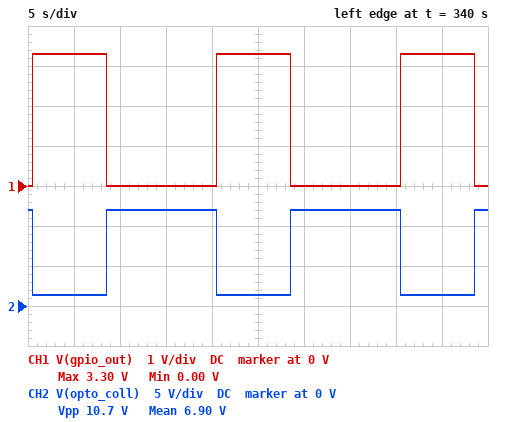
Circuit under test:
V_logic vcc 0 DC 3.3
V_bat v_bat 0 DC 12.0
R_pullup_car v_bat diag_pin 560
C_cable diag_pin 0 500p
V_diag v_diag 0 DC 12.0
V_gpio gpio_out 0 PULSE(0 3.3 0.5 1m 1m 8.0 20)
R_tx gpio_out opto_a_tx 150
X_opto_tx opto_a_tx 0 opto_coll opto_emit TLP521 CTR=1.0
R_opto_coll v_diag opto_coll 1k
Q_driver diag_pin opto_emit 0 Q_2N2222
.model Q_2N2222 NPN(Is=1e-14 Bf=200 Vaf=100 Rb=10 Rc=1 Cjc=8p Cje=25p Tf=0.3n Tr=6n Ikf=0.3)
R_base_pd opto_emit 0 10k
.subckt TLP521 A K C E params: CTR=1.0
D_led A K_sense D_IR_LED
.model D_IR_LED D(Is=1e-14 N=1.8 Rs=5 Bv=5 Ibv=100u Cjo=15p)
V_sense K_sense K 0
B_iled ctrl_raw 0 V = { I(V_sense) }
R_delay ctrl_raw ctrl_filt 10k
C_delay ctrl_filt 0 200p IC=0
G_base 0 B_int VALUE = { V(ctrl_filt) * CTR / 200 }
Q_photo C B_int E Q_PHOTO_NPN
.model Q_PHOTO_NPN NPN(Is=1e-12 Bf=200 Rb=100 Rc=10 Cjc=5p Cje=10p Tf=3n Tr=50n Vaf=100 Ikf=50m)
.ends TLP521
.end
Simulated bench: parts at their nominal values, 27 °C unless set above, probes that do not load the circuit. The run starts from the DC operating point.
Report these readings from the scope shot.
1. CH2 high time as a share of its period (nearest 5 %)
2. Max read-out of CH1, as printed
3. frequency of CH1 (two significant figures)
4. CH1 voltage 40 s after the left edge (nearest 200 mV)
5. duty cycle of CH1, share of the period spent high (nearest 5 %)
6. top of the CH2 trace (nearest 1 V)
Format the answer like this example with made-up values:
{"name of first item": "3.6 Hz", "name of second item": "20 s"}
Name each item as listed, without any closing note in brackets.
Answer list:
{"CH2 high time as a share of its period": "60 %", "Max read-out of CH1, as printed": "3.30 V", "frequency of CH1": "50 mHz", "CH1 voltage 40 s after the left edge": "0 V", "duty cycle of CH1, share of the period spent high": "40 %", "top of the CH2 trace": "12 V"}
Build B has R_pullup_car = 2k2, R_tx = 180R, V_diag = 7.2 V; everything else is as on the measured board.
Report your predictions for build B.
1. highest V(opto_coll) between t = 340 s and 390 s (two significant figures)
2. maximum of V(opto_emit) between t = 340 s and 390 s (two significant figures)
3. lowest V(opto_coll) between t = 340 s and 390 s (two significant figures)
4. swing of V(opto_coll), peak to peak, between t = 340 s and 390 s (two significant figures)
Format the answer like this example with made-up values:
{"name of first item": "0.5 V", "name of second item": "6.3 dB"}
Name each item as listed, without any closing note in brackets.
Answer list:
{"highest V(opto_coll) between t = 340 s and 390 s": "7.2 V", "maximum of V(opto_emit) between t = 340 s and 390 s": "790 mV", "lowest V(opto_coll) between t = 340 s and 390 s": "1.0 V", "swing of V(opto_coll), peak to peak, between t = 340 s and 390 s": "6.2 V"}
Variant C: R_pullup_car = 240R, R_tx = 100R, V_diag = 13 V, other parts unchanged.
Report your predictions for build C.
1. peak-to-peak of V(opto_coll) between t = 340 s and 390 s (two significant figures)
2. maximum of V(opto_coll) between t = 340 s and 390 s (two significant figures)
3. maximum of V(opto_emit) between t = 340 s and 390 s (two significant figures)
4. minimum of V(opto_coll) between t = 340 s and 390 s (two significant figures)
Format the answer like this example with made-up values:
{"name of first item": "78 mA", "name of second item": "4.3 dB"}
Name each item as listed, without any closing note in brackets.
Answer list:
{"peak-to-peak of V(opto_coll) between t = 340 s and 390 s": "12 V", "maximum of V(opto_coll) between t = 340 s and 390 s": "13 V", "maximum of V(opto_emit) between t = 340 s and 390 s": "890 mV", "minimum of V(opto_coll) between t = 340 s and 390 s": "1.2 V"}
